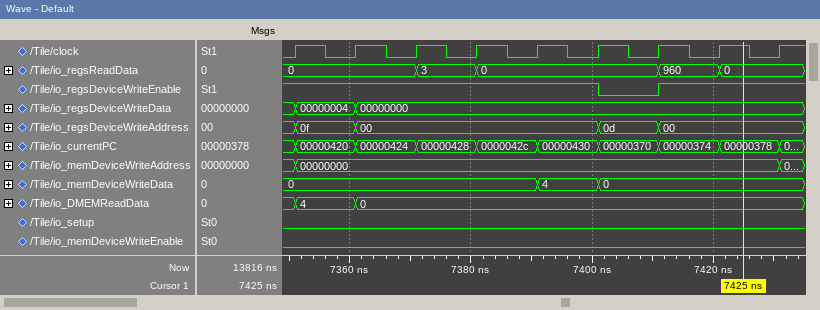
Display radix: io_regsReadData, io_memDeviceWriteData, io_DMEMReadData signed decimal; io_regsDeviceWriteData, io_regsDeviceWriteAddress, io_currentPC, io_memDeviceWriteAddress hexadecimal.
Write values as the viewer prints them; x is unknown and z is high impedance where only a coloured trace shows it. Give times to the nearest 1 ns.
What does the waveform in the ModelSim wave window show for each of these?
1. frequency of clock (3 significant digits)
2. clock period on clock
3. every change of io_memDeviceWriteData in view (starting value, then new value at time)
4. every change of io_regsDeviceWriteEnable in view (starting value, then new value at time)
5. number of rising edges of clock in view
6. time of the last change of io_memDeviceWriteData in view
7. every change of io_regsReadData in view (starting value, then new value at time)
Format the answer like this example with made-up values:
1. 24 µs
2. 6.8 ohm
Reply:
1. 100 MHz
2. 10 ns
3. 0, 4 at 7391 ns, 0 at 7401 ns
4. 1, 0 at 7401 ns, 1 at 7411 ns
5. 9
6. 7401 ns
7. 0, 3 at 7371 ns, 0 at 7381 ns, 960 at 7411 ns, 0 at 7421 ns
